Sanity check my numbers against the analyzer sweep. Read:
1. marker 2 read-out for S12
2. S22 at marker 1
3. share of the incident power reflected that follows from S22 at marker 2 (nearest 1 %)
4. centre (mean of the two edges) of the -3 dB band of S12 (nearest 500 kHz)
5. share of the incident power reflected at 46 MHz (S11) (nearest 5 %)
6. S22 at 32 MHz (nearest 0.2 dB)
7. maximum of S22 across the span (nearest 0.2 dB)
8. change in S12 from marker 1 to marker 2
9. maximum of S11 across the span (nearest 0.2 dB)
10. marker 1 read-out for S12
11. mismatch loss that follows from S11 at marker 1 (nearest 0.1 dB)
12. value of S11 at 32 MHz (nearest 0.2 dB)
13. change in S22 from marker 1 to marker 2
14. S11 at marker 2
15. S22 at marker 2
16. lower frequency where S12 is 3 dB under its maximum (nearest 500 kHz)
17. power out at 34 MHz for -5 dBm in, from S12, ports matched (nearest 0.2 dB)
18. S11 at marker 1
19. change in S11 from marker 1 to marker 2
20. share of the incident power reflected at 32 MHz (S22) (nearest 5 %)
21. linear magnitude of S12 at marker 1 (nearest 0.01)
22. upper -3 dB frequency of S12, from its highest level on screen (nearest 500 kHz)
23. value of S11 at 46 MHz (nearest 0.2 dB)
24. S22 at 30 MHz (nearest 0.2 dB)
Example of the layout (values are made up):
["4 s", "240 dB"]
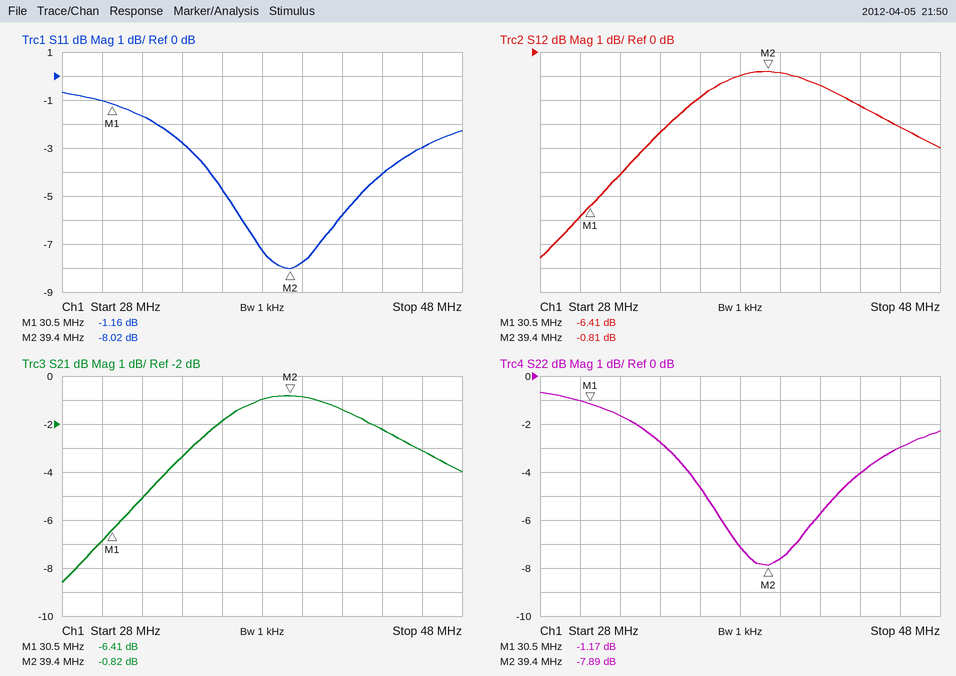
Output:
["-0.81 dB", "-1.17 dB", "16 %", "40.5 MHz", "50 %", "-1.6 dB", "-0.6 dB", "5.60 dB", "-0.6 dB", "-6.41 dB", "6.3 dB", "-1.6 dB", "-6.72 dB", "-8.02 dB", "-7.89 dB", "33.5 MHz", "-8.4 dBm", "-1.16 dB", "-6.86 dB", "70 %", "0.48", "47.5 MHz", "-3.0 dB", "-1.0 dB"]
